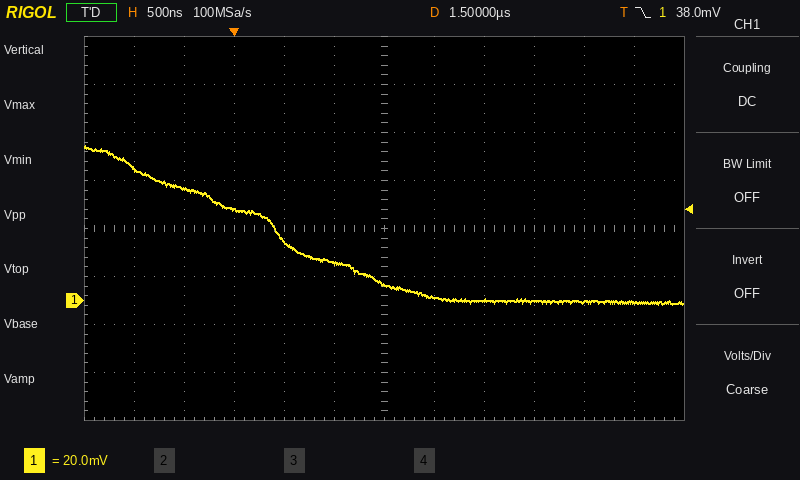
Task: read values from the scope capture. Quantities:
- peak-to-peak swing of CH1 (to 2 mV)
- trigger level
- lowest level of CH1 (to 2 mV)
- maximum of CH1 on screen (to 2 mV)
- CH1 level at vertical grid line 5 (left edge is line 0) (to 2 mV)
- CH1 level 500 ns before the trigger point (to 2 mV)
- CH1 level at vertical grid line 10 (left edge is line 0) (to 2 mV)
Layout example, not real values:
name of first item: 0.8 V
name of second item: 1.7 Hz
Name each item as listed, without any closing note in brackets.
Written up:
peak-to-peak swing of CH1: 66 mV
trigger level: 38.0 mV
lowest level of CH1: -2 mV
maximum of CH1 on screen: 64 mV
CH1 level at vertical grid line 5 (left edge is line 0): 16 mV
CH1 level 500 ns before the trigger point: 46 mV
CH1 level at vertical grid line 10 (left edge is line 0): 0 mV
